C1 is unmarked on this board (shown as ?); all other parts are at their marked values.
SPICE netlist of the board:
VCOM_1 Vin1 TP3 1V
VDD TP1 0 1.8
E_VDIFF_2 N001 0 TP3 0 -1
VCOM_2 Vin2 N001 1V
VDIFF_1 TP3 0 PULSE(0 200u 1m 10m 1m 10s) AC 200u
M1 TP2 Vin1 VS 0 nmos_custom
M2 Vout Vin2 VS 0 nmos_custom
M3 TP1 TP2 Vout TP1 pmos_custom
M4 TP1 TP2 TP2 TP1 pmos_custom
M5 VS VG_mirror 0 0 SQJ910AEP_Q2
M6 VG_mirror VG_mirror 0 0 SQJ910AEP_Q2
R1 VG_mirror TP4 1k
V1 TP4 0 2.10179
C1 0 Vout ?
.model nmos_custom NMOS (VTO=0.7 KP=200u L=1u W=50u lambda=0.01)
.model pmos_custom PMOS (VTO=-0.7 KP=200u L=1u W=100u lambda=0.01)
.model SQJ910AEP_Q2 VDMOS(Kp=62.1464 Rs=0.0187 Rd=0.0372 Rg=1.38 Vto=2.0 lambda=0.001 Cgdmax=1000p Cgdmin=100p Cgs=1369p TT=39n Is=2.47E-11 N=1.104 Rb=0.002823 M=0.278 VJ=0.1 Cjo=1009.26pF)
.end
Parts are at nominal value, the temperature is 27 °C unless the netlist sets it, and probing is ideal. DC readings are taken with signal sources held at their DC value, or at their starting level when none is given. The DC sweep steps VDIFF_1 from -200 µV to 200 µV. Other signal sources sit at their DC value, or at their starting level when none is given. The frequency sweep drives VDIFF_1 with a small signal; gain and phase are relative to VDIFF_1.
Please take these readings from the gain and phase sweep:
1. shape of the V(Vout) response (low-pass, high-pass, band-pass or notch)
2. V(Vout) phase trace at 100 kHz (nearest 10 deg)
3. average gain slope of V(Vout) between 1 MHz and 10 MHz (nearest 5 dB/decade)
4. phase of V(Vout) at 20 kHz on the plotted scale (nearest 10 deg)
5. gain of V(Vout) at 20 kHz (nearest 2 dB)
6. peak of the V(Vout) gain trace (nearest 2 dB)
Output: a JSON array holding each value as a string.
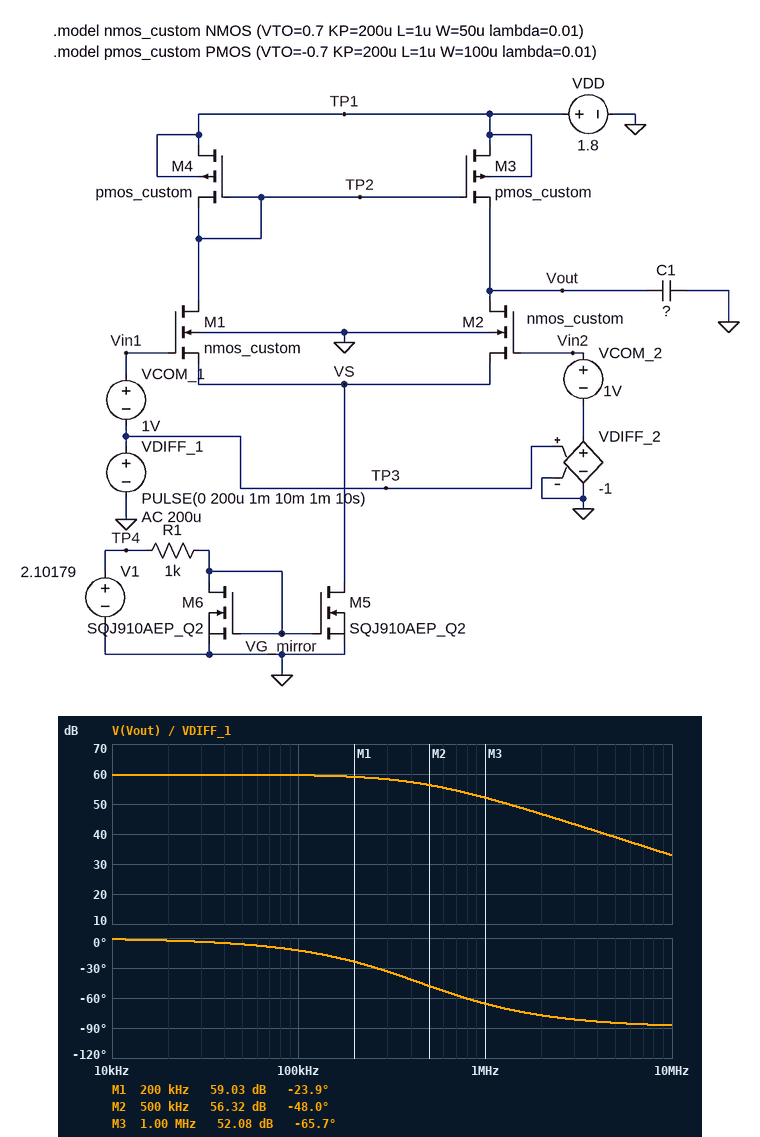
["low-pass", "-10 deg", "-20 dB/decade", "0 deg", "60 dB", "60 dB"]
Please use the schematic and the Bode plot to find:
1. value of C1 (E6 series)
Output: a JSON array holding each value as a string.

["1.5 pF"]
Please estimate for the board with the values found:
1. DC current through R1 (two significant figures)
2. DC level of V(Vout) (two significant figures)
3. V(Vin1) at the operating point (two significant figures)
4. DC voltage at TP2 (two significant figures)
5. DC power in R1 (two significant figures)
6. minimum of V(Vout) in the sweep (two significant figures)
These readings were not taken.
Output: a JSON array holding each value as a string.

["430 µA", "950 mV", "1.0 V", "950 mV", "180 µW", "760 mV"]
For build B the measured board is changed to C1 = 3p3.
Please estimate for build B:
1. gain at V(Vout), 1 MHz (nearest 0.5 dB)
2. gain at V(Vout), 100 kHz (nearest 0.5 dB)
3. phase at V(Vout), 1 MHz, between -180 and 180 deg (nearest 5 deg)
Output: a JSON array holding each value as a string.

["46.0 dB", "59.0 dB", "-80 deg"]
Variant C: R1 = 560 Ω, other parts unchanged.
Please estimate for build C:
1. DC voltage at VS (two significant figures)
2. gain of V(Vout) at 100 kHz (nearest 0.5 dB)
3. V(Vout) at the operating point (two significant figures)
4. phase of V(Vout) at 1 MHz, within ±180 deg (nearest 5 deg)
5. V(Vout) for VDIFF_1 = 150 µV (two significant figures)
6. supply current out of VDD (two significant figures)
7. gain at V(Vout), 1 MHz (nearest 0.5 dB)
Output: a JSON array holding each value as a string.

["33 mV", "57.5 dB", "910 mV", "-55 deg", "1.0 V", "720 µA", "53.0 dB"]
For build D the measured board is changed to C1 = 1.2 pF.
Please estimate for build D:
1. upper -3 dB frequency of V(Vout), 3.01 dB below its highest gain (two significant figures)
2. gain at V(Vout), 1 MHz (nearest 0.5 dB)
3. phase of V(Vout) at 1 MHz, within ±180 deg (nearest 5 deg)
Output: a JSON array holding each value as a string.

["560 kHz", "53.5 dB", "-60 deg"]
